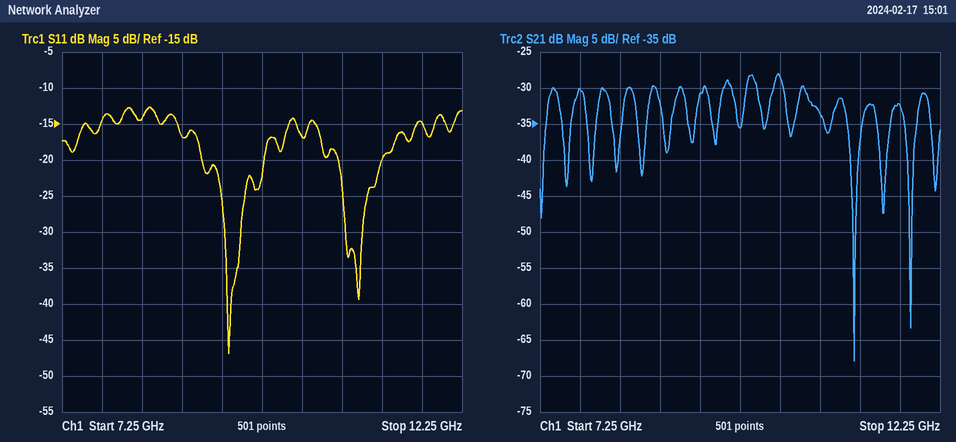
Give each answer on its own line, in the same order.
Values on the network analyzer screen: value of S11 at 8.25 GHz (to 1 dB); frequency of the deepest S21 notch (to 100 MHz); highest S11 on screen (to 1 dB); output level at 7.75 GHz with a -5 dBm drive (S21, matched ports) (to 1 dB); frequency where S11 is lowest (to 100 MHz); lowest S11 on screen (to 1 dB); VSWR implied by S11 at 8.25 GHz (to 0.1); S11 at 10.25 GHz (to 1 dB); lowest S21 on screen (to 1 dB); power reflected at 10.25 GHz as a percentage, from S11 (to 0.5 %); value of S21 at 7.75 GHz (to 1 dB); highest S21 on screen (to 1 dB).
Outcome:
-14 dB
11.2 GHz
-13 dB
-35 dBm
9.3 GHz
-47 dB
1.5
-17 dB
-68 dB
2.0 %
-30 dB
-28 dB
